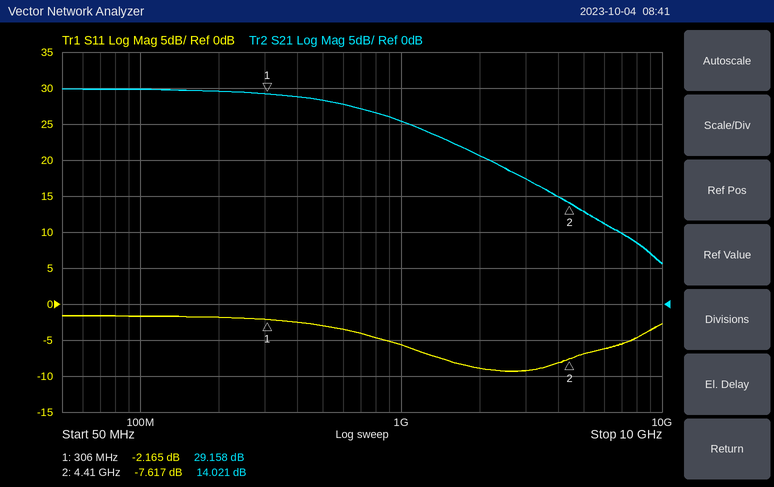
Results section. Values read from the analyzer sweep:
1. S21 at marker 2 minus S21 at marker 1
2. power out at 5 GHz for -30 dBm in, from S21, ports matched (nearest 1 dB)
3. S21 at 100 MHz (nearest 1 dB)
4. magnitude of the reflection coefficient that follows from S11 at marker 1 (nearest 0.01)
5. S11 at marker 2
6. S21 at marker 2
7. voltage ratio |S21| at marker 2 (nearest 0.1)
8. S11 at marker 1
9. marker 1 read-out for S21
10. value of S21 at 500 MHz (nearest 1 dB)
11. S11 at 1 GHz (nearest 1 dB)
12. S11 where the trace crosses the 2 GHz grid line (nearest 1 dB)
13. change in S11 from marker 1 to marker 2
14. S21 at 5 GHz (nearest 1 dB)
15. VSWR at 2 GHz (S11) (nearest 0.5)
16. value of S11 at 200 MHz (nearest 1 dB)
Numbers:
-15.137 dB
-17 dBm
30 dB
0.78
-7.617 dB
14.021 dB
5.0
-2.165 dB
29.158 dB
28 dB
-6 dB
-9 dB
-5.452 dB
13 dB
2.0
-2 dB
